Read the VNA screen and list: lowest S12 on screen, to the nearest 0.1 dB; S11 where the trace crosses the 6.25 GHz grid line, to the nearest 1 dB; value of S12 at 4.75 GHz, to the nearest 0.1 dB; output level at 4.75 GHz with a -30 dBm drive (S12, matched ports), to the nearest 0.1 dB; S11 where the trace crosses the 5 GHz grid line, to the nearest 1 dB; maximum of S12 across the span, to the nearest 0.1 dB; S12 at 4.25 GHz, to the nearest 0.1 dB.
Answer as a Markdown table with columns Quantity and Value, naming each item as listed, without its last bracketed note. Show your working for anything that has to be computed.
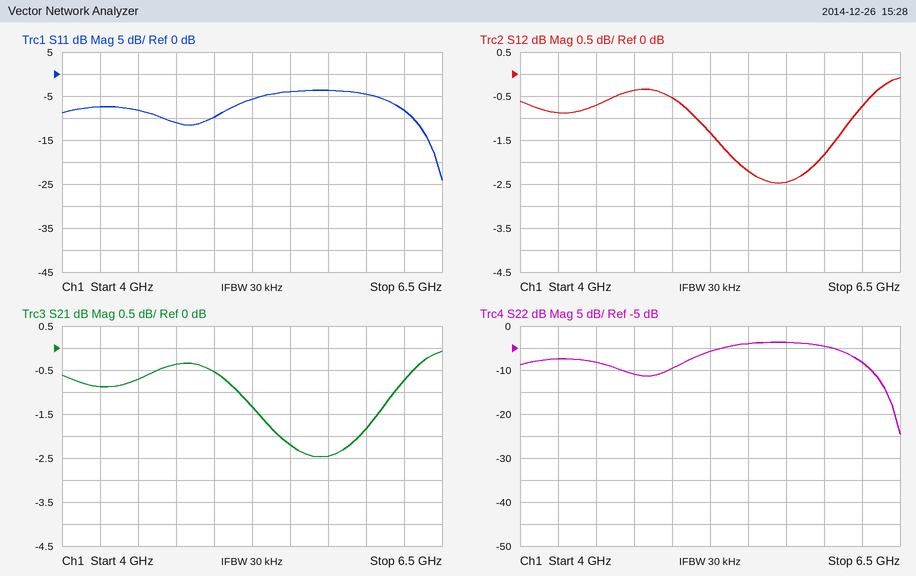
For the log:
| Quantity | Value |
|---|---|
| lowest S12 on screen, to the nearest 0.1 dB | -2.5 dB |
| S11 where the trace crosses the 6.25 GHz grid line, to the nearest 1 dB | -8 dB |
| value of S12 at 4.75 GHz, to the nearest 0.1 dB | -0.4 dB |
| output level at 4.75 GHz with a -30 dBm drive (S12, matched ports), to the nearest 0.1 dB | -30 dBm + (-0.4 dB) = -30.4 dBm |
| S11 where the trace crosses the 5 GHz grid line, to the nearest 1 dB | -10 dB |
| maximum of S12 across the span, to the nearest 0.1 dB | -0.1 dB |
| S12 at 4.25 GHz, to the nearest 0.1 dB | -0.9 dB |
